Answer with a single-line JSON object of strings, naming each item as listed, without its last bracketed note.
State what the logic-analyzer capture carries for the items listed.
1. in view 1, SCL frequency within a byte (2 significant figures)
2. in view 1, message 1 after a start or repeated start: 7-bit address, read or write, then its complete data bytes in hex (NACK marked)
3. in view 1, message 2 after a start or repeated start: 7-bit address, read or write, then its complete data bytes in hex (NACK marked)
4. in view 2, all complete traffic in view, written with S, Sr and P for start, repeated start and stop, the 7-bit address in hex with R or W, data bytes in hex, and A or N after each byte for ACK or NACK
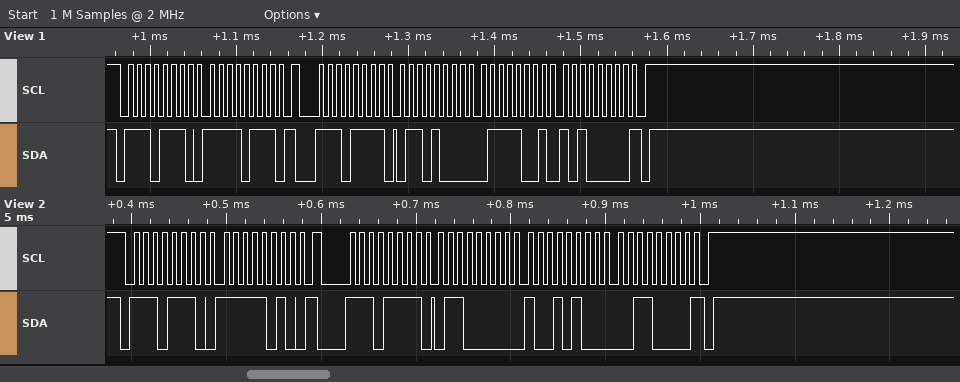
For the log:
{"in view 1, SCL frequency within a byte": "100 kHz", "in view 1, message 1 after a start or repeated start: 7-bit address, read or write, then its complete data bytes in hex": "0x77 write: F7", "in view 1, message 2 after a start or repeated start: 7-bit address, read or write, then its complete data bytes in hex": "0x77 read: 68 79 A0 NACK", "in view 2, all complete traffic in view, written with S, Sr and P for start, repeated start and stop, the 7-bit address in hex with R or W, data bytes in hex, and A or N after each byte for ACK or NACK": "S 77W A FA A Sr 77R A 60 A 94 A 30 N P"}
